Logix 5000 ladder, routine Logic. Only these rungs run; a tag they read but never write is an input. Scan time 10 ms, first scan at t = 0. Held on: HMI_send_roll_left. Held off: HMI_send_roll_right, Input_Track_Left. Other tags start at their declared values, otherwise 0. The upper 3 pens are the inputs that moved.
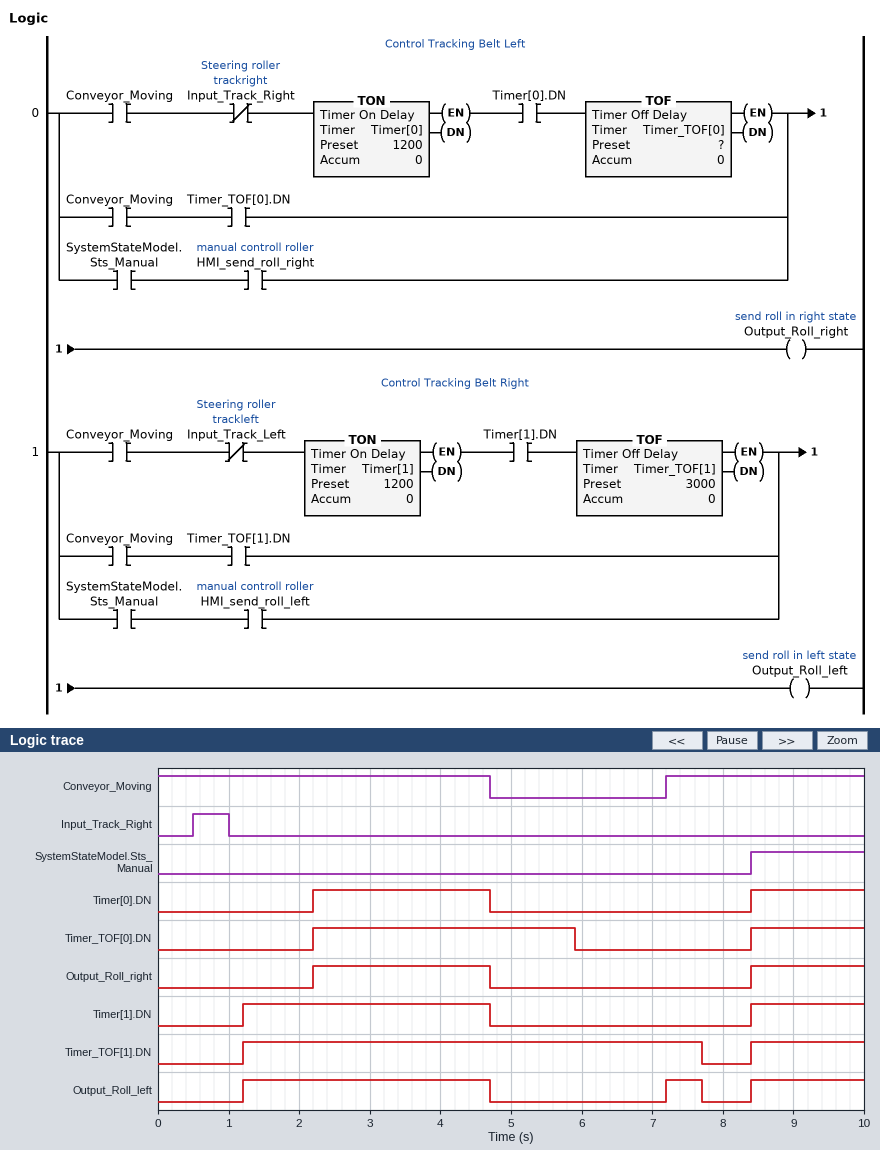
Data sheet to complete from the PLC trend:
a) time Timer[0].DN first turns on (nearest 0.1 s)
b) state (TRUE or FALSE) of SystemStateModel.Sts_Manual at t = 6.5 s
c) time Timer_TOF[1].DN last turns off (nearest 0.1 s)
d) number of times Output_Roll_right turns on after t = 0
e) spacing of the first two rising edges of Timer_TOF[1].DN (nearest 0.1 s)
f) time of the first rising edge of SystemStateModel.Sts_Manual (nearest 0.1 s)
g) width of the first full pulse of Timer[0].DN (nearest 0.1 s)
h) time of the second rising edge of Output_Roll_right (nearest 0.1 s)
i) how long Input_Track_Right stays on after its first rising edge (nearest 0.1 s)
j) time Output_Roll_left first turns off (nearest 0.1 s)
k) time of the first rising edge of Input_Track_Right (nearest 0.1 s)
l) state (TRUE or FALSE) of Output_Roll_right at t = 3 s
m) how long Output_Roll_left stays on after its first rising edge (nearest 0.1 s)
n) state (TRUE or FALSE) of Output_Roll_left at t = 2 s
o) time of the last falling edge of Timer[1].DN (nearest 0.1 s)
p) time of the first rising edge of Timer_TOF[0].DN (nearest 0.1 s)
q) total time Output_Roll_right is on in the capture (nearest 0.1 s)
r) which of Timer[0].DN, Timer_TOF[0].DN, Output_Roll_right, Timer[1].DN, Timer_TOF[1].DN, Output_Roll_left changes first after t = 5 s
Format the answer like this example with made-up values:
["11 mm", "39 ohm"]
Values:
["2.2 s", "FALSE", "7.7 s", "2", "7.2 s", "8.4 s", "2.5 s", "8.4 s", "0.5 s", "4.7 s", "0.5 s", "TRUE", "3.5 s", "TRUE", "4.7 s", "2.2 s", "4.1 s", "Timer_TOF[0].DN"]
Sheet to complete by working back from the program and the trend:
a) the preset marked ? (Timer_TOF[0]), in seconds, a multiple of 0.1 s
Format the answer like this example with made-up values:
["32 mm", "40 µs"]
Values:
["1.2 s"]
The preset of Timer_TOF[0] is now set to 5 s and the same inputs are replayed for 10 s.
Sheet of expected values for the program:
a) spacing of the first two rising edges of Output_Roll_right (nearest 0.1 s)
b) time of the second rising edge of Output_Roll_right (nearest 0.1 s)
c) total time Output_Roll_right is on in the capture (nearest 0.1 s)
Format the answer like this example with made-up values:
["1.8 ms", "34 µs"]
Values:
["5.0 s", "7.2 s", "5.3 s"]
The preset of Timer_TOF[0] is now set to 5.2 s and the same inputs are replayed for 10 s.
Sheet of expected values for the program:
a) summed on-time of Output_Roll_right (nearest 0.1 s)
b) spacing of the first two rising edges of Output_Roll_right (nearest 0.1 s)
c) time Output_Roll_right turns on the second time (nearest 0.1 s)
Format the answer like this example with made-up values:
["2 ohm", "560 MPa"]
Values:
["5.3 s", "5.0 s", "7.2 s"]
